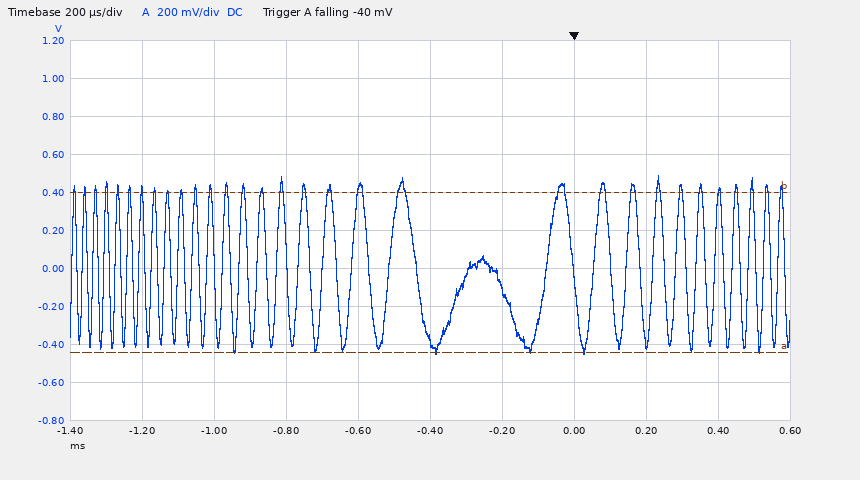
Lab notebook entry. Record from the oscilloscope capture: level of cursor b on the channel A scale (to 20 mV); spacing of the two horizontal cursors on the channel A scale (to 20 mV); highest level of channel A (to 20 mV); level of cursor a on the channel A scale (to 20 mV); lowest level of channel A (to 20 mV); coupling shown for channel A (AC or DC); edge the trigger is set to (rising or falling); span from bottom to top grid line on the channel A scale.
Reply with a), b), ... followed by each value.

a) 400 mV
b) 840 mV
c) 480 mV
d) -440 mV
e) -440 mV
f) DC
g) falling
h) 2 V
